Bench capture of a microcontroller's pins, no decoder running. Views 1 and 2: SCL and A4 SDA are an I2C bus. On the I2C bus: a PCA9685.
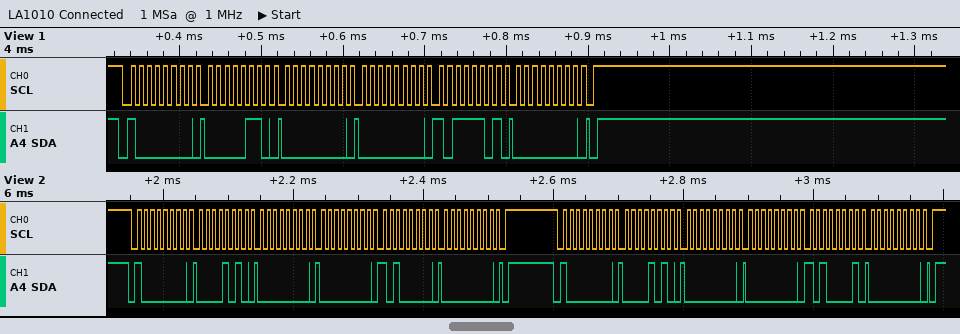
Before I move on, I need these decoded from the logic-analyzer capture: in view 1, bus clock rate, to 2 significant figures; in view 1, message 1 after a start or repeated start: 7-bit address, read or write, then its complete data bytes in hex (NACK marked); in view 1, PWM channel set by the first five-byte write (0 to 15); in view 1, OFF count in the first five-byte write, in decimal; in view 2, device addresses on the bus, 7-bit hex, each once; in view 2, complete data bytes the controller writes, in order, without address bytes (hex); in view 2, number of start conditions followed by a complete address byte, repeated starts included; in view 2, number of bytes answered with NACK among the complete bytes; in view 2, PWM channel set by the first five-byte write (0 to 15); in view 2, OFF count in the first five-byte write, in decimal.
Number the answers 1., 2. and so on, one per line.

1. 100 kHz
2. 0x40 write: 06 00 00 BD 00
3. 0
4. 189
5. 0x40
6. 0A 00 00 A0 00 0A 00 00 A1 00
7. 2
8. 0
9. 1
10. 160
